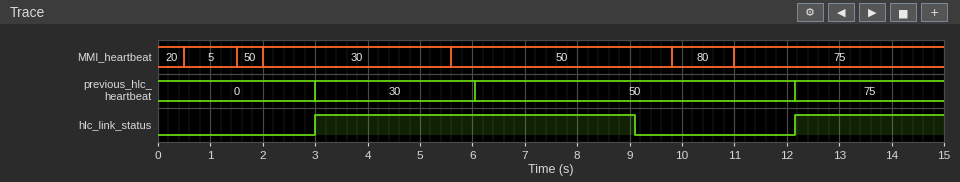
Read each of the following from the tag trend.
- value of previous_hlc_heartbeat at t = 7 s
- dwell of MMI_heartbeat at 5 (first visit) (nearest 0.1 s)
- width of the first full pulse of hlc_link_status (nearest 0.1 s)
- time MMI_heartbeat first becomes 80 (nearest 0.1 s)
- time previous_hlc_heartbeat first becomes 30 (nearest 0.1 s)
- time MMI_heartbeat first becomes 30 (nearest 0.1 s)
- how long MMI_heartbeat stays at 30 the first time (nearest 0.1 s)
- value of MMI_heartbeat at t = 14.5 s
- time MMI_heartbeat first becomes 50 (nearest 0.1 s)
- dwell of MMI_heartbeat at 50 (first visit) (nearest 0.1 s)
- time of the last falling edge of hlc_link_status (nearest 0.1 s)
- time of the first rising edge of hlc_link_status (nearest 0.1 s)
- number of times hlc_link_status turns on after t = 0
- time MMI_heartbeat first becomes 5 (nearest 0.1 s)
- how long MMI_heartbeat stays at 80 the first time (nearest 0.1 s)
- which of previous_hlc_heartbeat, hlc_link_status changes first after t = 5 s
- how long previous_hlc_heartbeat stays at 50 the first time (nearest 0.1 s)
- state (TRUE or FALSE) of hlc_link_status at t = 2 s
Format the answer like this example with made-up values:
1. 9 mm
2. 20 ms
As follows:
1. 50
2. 1.0 s
3. 6.1 s
4. 9.8 s
5. 3.0 s
6. 2.0 s
7. 3.6 s
8. 75
9. 1.5 s
10. 0.5 s
11. 9.1 s
12. 3.0 s
13. 2
14. 0.5 s
15. 1.2 s
16. previous_hlc_heartbeat
17. 6.1 s
18. FALSE
